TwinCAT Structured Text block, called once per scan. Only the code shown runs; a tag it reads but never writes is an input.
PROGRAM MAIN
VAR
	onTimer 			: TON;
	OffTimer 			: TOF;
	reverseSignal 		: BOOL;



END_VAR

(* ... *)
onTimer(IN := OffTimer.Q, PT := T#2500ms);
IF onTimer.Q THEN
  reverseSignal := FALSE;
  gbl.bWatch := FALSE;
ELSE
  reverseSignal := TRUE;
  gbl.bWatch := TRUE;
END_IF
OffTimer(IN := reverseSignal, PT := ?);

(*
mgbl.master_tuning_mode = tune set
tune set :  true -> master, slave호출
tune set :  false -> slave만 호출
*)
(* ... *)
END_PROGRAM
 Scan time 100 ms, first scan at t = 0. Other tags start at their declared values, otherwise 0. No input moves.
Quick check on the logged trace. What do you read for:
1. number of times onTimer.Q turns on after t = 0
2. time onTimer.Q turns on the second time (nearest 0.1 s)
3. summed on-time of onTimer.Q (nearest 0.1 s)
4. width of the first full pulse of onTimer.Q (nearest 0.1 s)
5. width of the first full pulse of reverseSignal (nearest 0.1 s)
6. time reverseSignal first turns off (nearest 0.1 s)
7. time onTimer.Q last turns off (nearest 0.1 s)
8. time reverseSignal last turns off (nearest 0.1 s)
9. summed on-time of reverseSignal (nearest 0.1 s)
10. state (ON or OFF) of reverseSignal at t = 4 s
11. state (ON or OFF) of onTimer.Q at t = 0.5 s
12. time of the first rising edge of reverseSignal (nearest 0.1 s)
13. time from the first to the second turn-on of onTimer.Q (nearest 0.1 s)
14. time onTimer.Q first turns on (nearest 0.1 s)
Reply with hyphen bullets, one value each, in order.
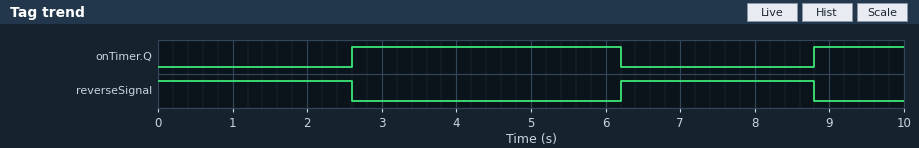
- 2
- 8.8 s
- 4.8 s
- 3.6 s
- 2.6 s
- 2.6 s
- 6.2 s
- 8.8 s
- 5.2 s
- OFF
- OFF
- 6.2 s
- 6.2 s
- 2.6 s
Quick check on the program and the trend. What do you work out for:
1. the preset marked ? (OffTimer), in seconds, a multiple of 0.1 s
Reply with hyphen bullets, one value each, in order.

- 3.5 s
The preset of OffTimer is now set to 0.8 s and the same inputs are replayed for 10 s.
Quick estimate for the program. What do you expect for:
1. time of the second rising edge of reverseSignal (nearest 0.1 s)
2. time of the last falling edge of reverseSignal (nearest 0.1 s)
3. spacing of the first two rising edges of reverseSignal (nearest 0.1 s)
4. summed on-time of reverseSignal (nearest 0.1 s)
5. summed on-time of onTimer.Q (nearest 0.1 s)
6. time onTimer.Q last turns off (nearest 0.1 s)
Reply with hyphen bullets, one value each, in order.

- 7.0 s
- 9.6 s
- 3.5 s
- 7.8 s
- 2.2 s
- 7.0 s
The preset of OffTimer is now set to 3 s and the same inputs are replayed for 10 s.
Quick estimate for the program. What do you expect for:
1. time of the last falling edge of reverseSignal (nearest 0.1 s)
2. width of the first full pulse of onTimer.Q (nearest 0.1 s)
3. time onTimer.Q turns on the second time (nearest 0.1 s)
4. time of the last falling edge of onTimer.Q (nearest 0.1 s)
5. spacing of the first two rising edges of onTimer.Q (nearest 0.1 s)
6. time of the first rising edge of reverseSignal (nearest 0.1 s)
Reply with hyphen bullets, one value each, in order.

- 8.3 s
- 3.1 s
- 8.3 s
- 5.7 s
- 5.7 s
- 5.7 s
